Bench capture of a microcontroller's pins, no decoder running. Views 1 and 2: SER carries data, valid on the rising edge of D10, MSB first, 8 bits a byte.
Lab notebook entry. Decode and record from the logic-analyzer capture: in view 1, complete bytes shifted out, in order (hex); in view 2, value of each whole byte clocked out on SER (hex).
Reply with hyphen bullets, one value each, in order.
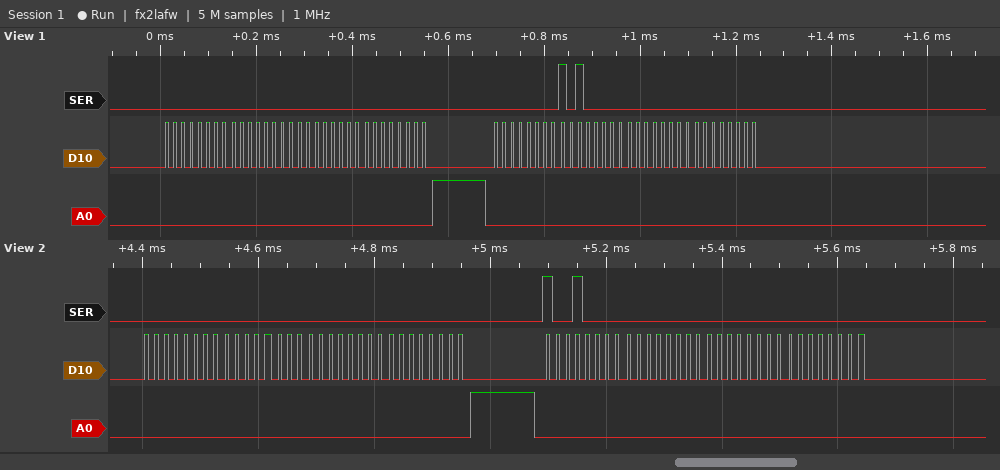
- 0x00 0x00 0x00 0x00 0x00 0xA0 0x00 0x00
- 0x00 0x00 0x00 0x00 0x90 0x00 0x00 0x00
